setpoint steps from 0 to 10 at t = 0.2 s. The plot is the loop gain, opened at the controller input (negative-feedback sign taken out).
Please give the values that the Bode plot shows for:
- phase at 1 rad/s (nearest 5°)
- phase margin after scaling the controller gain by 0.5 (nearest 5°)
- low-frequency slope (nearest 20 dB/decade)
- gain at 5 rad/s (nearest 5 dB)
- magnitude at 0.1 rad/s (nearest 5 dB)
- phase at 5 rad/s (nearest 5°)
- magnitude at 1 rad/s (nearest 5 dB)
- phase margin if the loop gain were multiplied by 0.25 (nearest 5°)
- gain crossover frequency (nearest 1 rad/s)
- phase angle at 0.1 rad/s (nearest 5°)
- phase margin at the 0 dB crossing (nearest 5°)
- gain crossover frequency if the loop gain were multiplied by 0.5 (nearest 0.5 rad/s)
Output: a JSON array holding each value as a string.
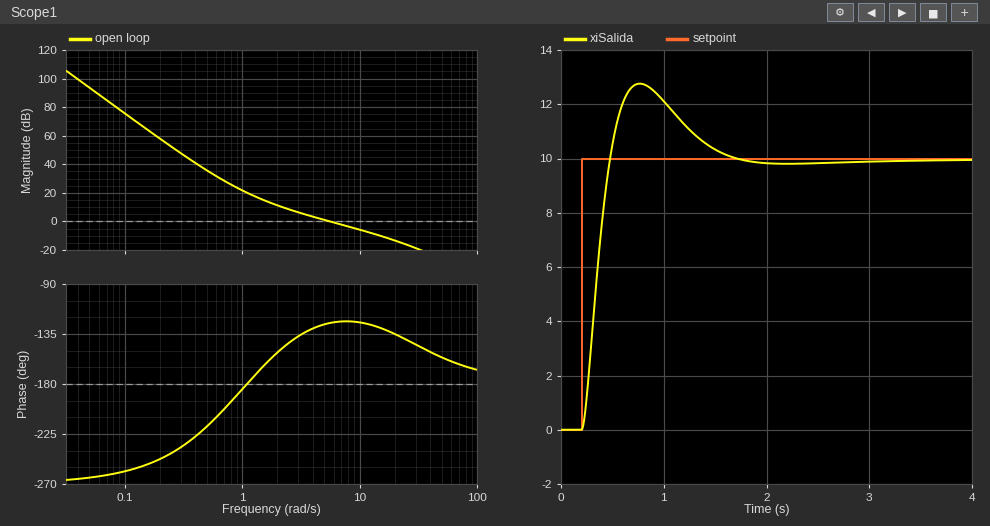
["-185°", "45°", "-60 dB/decade", "0 dB", "75 dB", "-125°", "20 dB", "25°", "6 rad/s", "-260°", "55°", "3.0 rad/s"]
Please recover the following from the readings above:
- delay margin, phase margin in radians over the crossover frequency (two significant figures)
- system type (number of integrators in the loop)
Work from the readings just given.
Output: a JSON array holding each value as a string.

["0.16 s", "3"]
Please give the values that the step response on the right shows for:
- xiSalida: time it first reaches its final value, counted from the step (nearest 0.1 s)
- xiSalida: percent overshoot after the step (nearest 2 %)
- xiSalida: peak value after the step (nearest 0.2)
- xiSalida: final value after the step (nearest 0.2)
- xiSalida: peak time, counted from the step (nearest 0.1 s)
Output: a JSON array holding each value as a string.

["0.3 s", "28 %", "12.8", "10.0", "0.6 s"]
